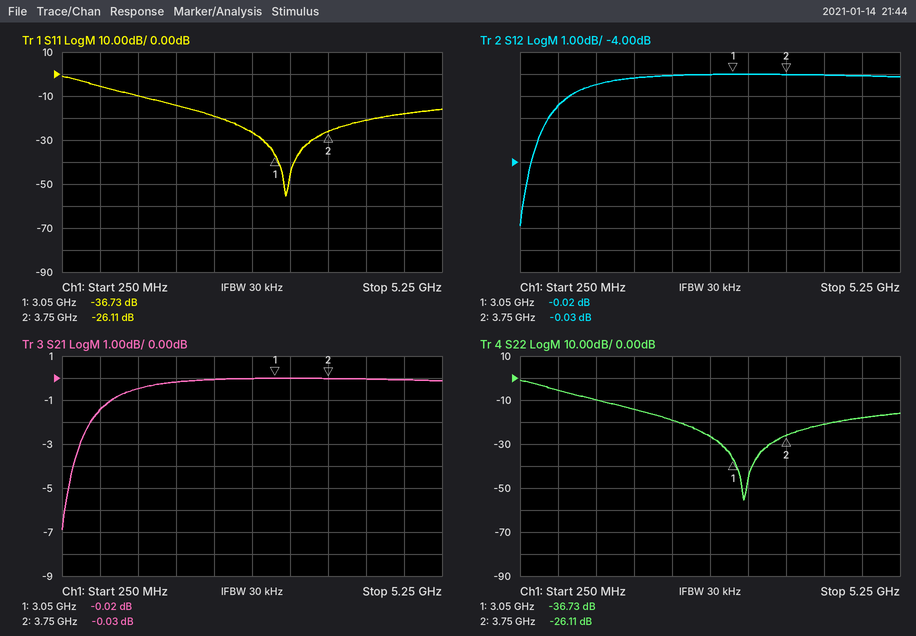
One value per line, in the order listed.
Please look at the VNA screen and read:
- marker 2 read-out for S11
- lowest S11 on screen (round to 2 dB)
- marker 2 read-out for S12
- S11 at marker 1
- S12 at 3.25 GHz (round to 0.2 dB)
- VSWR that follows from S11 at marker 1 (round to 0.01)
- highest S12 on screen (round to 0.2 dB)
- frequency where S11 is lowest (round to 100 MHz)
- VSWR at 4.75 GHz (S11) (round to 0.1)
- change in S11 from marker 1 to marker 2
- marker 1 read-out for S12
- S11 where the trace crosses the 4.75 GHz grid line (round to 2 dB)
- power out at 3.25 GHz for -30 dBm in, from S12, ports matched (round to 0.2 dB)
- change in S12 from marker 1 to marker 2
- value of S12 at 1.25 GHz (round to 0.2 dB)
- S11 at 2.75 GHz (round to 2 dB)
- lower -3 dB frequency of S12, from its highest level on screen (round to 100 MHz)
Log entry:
-26.11 dB
-56 dB
-0.03 dB
-36.73 dB
0.0 dB
1.03
0.0 dB
3.2 GHz
1.3
10.62 dB
-0.02 dB
-18 dB
-30.0 dBm
-0.01 dB
-0.4 dB
-26 dB
500 MHz
